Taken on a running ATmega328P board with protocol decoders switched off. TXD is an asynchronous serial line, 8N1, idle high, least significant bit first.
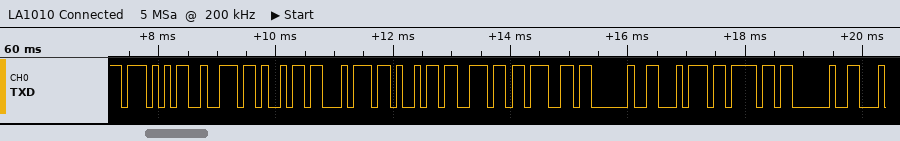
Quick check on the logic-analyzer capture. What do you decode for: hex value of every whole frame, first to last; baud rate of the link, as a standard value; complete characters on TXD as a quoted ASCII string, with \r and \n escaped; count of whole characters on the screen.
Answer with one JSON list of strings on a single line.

["0x57 0x72 0x69 0x74 0x69 0x6E 0x67 0x20 0x74 0x6F 0x20", "9600 baud", "\"Writing to \"", "11"]
